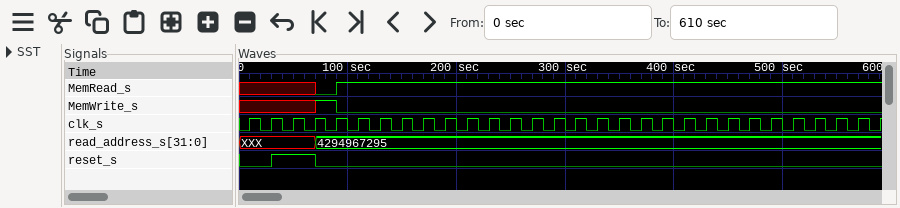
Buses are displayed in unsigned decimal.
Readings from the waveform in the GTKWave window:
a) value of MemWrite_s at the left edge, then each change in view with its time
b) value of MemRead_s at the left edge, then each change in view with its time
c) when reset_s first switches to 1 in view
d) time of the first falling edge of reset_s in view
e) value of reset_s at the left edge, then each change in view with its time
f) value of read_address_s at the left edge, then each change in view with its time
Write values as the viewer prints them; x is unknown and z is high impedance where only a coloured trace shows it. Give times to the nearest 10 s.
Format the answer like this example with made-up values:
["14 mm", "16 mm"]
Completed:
["x, 1 at 70 s, 0 at 90 s", "x, 0 at 70 s, 1 at 90 s", "30 s", "70 s", "0, 1 at 30 s, 0 at 70 s", "XXX, 4294967295 at 70 s"]
